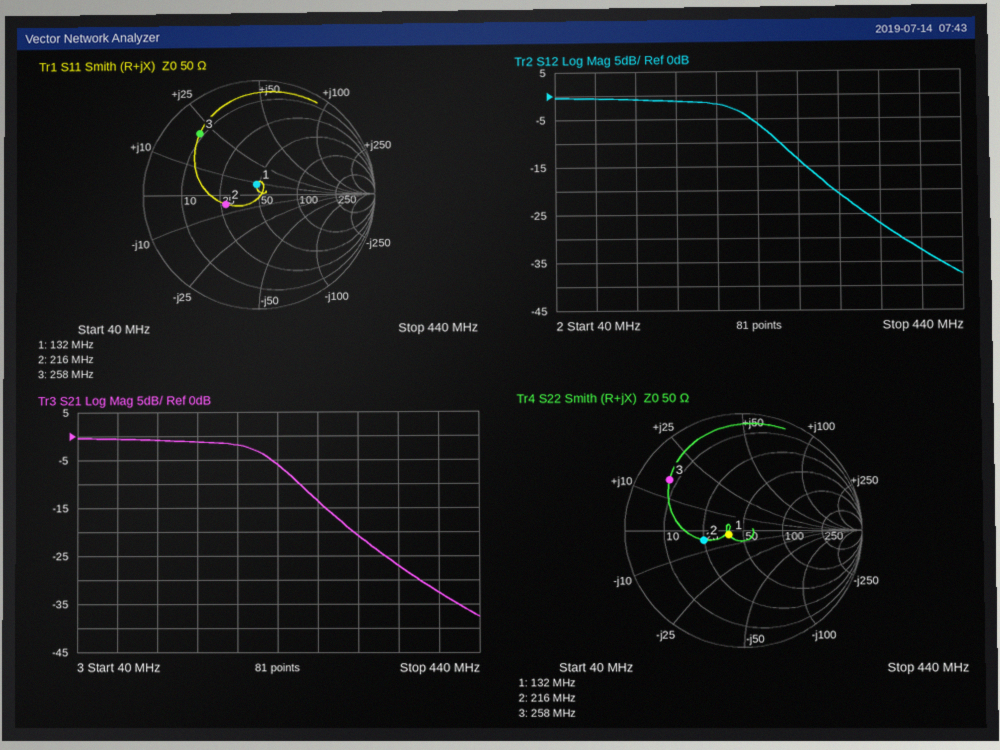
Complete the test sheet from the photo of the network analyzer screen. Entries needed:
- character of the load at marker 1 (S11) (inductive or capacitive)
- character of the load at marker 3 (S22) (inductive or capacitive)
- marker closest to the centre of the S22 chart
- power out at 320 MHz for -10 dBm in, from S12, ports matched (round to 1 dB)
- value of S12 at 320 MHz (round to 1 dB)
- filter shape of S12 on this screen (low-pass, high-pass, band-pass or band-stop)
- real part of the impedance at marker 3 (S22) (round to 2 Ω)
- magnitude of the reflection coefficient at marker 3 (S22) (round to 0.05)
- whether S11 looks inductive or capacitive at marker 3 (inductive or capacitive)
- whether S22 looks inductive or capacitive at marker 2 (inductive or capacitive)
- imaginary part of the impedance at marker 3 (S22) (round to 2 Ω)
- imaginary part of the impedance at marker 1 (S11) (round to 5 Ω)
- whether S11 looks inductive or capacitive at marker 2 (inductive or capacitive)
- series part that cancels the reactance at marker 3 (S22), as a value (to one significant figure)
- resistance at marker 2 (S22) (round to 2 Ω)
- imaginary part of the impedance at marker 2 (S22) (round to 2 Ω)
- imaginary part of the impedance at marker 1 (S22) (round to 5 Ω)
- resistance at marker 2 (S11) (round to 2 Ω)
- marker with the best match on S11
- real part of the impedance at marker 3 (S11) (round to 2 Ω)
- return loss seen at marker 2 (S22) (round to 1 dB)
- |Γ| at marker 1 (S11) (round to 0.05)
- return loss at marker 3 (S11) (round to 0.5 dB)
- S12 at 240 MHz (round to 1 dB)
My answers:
inductive
inductive
marker 1
-31 dBm
-21 dB
low-pass
8 Ω
0.75
inductive
capacitive
+16 Ω
+10 Ω
capacitive
40 pF
24 Ω
-4 Ω
-5 Ω
28 Ω
marker 1
8 Ω
9 dB
0.10
2.5 dB
-6 dB
